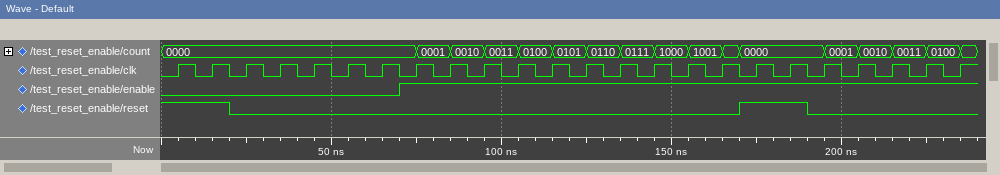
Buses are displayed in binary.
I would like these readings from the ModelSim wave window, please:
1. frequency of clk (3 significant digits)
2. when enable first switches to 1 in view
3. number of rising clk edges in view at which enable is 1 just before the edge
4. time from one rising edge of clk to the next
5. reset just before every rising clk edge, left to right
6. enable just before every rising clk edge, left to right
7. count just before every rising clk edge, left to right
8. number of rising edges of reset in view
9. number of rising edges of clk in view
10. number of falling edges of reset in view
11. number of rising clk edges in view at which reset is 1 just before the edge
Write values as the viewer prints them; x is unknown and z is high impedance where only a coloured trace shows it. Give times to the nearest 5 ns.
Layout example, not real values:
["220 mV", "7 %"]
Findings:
["100 MHz", "70 ns", "17", "10 ns", "1 1 0 0 0 0 0 0 0 0 0 0 0 0 0 0 0 1 1 0 0 0 0 0", "0 0 0 0 0 0 0 1 1 1 1 1 1 1 1 1 1 1 1 1 1 1 1 1", "0000, 0000, 0000, 0000, 0000, 0000, 0000, 0000, 0001, 0010, 0011, 0100, 0101, 0110, 0111, 1000, 1001, 0000, 0000, 0000, 0001, 0010, 0011, 0100", "1", "24", "2", "4"]
